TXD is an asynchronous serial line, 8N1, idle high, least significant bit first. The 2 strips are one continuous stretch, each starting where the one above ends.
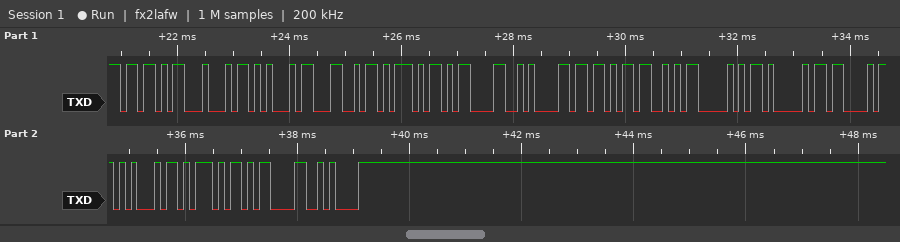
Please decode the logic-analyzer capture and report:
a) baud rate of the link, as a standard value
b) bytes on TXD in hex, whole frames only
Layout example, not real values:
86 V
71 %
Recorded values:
9600 baud
0x5B 0x44 0x45 0x4C 0x5D 0x0D 0x0A 0x5B 0x53 0x50 0x41 0x43 0x45 0x5D 0x0D 0x0A
